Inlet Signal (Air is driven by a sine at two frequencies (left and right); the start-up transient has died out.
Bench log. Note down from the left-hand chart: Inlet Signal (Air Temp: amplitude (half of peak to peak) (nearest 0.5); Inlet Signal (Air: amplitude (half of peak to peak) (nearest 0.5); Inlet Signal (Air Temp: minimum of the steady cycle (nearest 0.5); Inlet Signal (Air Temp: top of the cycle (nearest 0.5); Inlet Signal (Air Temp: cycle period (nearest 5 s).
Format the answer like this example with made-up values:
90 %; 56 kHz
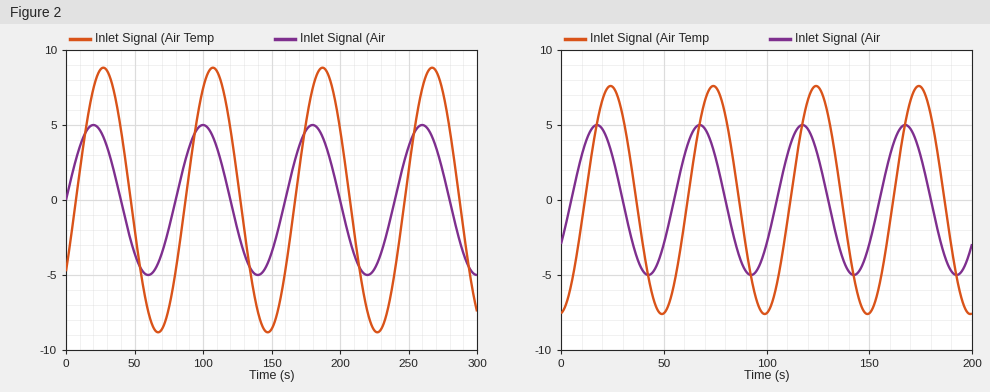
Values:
9.0; 5.0; -9.0; 9.0; 80 s
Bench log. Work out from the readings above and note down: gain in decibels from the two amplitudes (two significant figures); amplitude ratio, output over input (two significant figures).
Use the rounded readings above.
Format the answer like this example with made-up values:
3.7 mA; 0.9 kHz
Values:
5.1 dB; 1.8
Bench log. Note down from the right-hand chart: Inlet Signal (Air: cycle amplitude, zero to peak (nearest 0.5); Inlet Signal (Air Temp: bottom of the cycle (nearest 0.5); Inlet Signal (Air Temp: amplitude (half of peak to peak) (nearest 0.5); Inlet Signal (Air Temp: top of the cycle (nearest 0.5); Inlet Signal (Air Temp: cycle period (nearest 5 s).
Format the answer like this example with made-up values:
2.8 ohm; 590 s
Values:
5.0; -7.5; 7.5; 7.5; 50 s
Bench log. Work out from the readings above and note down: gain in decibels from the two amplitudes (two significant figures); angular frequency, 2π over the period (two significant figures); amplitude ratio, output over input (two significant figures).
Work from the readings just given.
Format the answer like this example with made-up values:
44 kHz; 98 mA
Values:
3.5 dB; 0.13 rad/s; 1.5
